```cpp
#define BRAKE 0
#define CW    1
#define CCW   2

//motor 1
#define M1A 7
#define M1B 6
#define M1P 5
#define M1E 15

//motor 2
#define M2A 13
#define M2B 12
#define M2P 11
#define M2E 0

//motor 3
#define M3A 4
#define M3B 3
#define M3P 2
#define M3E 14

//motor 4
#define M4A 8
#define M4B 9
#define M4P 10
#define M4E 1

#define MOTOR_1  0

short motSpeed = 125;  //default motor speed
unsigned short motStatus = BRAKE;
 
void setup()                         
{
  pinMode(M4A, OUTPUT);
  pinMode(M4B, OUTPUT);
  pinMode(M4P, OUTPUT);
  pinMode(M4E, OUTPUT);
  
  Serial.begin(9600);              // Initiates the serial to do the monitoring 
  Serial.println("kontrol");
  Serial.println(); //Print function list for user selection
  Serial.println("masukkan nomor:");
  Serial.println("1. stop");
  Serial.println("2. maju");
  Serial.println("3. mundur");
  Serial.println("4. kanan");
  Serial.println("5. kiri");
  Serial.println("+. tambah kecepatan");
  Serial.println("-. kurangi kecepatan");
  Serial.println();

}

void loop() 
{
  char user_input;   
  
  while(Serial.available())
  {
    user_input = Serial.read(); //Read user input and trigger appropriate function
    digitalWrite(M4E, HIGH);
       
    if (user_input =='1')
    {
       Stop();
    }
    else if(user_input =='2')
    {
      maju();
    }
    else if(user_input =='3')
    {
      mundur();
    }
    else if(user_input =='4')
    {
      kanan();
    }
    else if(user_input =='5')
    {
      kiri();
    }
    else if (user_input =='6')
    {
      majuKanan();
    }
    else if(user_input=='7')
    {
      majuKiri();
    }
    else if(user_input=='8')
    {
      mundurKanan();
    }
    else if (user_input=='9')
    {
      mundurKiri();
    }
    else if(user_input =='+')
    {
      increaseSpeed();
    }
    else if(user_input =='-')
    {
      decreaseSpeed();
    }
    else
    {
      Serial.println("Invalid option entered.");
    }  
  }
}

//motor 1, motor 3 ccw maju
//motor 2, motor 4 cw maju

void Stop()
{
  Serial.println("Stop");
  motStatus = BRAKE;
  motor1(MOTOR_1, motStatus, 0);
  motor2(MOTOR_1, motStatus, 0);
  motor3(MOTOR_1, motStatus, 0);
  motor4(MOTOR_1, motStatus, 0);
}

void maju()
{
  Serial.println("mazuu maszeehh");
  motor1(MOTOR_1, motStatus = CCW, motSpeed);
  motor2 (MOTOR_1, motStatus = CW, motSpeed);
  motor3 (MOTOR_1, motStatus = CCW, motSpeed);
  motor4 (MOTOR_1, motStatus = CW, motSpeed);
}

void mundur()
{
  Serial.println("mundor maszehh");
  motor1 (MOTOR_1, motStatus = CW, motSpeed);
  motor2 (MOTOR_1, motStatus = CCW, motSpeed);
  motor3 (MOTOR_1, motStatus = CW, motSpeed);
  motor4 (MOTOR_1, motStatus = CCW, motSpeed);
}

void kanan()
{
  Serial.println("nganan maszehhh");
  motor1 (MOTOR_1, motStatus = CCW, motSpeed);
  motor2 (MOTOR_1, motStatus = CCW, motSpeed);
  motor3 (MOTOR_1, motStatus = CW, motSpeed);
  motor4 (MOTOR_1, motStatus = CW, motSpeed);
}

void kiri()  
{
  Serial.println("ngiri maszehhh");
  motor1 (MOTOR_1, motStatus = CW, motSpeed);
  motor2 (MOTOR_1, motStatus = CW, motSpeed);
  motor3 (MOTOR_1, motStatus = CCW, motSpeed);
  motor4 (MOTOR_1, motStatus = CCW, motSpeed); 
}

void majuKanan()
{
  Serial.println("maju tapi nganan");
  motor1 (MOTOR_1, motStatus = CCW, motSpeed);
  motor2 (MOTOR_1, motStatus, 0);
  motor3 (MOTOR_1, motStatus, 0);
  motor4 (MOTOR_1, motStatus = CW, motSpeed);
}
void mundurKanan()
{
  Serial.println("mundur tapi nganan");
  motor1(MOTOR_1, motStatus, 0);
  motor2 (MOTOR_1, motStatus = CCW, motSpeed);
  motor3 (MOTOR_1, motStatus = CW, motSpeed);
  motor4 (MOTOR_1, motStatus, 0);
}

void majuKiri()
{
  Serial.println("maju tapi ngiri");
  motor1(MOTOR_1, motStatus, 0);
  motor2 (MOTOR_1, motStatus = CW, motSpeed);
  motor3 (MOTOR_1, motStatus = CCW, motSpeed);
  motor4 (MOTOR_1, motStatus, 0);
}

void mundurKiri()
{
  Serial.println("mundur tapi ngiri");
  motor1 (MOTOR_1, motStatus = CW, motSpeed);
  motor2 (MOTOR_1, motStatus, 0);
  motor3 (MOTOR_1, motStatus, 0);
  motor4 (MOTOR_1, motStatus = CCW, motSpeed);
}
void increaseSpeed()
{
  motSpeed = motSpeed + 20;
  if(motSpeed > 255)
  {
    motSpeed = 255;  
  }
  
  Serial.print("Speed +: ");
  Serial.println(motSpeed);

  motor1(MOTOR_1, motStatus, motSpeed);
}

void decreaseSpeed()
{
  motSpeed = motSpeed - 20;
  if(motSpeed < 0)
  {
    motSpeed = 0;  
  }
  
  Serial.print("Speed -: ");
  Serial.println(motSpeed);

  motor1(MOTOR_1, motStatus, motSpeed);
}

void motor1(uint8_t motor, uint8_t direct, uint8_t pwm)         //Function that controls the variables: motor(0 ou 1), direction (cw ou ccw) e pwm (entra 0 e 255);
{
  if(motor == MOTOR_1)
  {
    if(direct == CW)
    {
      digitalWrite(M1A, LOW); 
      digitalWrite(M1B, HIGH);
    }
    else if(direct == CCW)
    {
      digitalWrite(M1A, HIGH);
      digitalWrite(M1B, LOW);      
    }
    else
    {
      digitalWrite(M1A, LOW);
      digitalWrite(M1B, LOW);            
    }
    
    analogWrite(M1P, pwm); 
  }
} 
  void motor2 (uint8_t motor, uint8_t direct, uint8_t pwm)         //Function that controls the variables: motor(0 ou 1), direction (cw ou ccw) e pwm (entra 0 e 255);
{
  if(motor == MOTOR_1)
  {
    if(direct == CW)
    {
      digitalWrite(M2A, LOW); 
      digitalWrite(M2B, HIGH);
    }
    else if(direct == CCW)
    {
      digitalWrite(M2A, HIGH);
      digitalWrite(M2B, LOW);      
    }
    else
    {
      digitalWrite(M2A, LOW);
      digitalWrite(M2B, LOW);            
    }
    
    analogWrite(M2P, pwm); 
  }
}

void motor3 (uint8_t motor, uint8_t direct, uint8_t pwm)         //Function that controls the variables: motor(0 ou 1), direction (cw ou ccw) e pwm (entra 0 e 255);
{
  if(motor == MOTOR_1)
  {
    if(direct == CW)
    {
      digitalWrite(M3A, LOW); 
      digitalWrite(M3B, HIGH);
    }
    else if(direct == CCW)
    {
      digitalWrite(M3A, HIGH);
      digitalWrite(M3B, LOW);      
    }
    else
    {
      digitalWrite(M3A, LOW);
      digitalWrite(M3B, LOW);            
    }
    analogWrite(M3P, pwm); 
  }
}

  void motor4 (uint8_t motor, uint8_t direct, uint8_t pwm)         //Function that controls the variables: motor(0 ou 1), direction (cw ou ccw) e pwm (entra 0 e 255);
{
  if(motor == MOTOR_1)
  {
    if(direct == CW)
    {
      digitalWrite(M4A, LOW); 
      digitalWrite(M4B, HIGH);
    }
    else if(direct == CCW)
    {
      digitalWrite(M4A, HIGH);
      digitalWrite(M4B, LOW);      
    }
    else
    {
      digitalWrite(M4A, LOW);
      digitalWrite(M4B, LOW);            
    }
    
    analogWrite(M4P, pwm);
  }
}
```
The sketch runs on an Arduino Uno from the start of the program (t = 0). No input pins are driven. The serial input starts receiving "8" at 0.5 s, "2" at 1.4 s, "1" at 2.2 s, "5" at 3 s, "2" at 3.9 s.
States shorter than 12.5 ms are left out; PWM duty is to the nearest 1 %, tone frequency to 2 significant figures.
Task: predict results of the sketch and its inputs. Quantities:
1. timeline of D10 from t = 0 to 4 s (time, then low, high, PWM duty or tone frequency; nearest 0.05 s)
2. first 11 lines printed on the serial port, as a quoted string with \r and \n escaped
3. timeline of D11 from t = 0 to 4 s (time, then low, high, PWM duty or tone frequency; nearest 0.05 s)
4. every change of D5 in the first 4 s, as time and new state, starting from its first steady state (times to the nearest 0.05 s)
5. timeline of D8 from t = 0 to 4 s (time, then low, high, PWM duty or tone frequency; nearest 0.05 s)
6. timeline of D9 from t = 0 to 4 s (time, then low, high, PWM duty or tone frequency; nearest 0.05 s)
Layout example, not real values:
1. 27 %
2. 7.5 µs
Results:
1. 0 s low; 1.4 s PWM 49 %; 2.2 s low; 3 s PWM 49 %
2. "kontrol\r\n\r\nmasukkan nomor:\r\n1. stop\r\n2. maju\r\n3. mundur\r\n4. kanan\r\n5. kiri\r\n+. tambah kecepatan\r\n-. kurangi kecepatan\r\n\r\n"
3. 0.5 s PWM 49 %; 2.2 s low; 3 s PWM 49 %
4. 0.5 s low; 1.4 s PWM 49 %; 2.2 s low; 3 s PWM 49 %
5. 0 s low; 3 s high; 3.9 s low
6. 0 s low; 0.5 s high; 2.2 s low; 3.9 s high
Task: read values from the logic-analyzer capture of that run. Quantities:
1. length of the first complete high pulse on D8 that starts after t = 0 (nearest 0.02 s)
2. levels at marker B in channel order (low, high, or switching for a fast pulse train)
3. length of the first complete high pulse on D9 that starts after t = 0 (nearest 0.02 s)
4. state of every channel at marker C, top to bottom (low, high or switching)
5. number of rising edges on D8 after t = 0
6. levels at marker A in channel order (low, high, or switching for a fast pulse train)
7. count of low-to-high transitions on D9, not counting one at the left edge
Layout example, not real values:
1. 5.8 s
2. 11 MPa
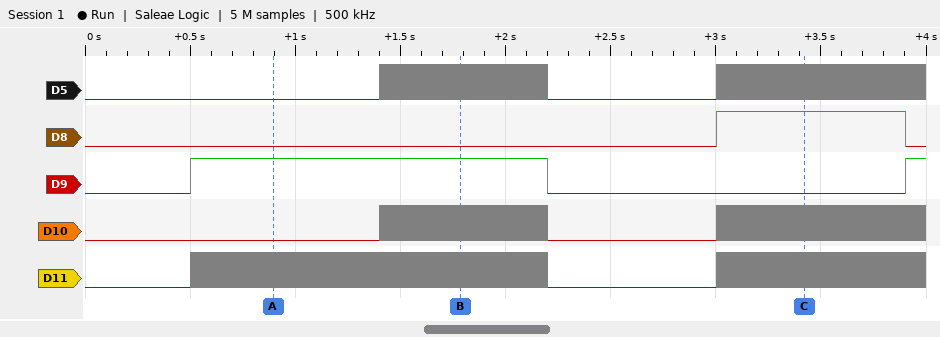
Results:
1. 0.90 s
2. D5 switching, D8 low, D9 high, D10 switching, D11 switching
3. 1.70 s
4. D5 switching, D8 high, D9 low, D10 switching, D11 switching
5. 1
6. D5 low, D8 low, D9 high, D10 low, D11 switching
7. 2
